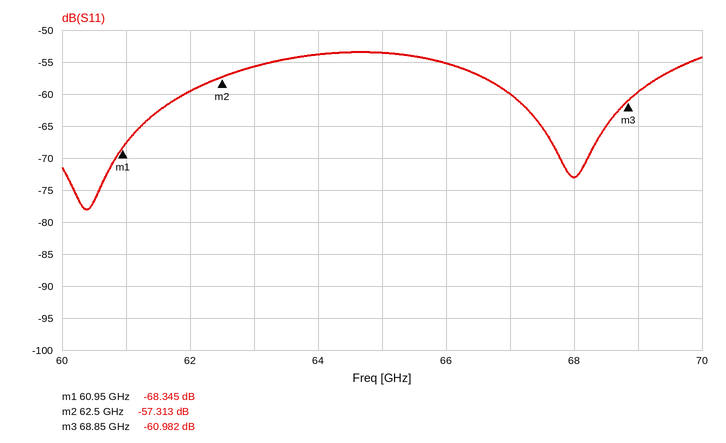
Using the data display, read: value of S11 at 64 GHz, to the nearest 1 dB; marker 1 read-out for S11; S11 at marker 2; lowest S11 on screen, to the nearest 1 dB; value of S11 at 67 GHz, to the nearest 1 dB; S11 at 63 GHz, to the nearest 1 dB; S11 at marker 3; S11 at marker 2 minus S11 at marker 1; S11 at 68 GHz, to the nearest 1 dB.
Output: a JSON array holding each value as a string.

["-54 dB", "-68.345 dB", "-57.313 dB", "-78 dB", "-60 dB", "-56 dB", "-60.982 dB", "11.032 dB", "-73 dB"]
